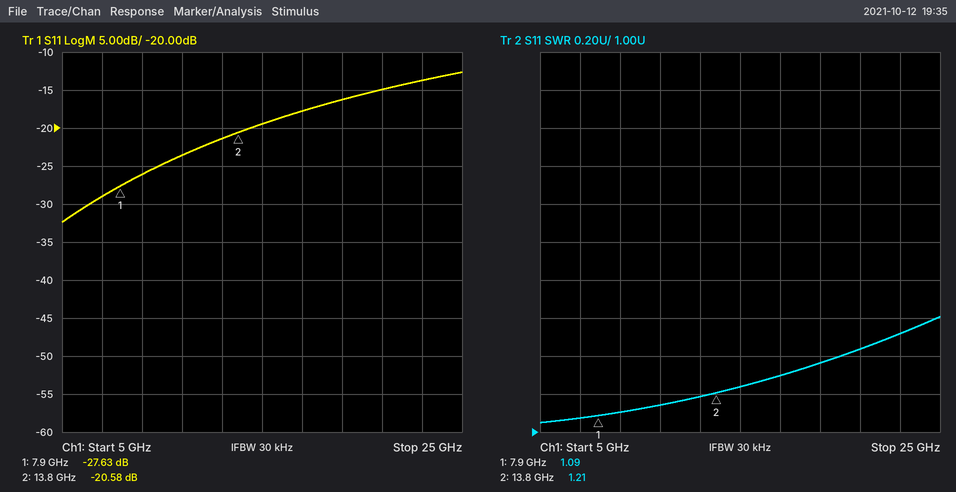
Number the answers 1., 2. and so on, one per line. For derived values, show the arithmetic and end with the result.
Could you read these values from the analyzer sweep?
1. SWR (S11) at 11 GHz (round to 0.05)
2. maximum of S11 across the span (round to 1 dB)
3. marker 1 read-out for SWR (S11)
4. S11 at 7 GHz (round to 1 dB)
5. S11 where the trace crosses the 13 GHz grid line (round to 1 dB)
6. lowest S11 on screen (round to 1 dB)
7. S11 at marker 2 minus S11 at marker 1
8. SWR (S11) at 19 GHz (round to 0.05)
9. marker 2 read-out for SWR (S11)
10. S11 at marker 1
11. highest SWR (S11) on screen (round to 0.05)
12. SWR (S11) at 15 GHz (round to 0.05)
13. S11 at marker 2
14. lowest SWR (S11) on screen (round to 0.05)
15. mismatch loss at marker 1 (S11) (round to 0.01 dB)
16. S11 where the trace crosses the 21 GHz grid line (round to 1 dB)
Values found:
1. 1.15
2. -13 dB
3. 1.09
4. -29 dB
5. -21 dB
6. -32 dB
7. -20.58 − (-27.63) = 7.05 dB
8. 1.35
9. 1.21
10. -27.63 dB
11. 1.60
12. 1.25
13. -20.58 dB
14. 1.05
15. −10 log10(1 − 10^(-27.63/10)) ≈ 0.01 dB
16. -15 dB
